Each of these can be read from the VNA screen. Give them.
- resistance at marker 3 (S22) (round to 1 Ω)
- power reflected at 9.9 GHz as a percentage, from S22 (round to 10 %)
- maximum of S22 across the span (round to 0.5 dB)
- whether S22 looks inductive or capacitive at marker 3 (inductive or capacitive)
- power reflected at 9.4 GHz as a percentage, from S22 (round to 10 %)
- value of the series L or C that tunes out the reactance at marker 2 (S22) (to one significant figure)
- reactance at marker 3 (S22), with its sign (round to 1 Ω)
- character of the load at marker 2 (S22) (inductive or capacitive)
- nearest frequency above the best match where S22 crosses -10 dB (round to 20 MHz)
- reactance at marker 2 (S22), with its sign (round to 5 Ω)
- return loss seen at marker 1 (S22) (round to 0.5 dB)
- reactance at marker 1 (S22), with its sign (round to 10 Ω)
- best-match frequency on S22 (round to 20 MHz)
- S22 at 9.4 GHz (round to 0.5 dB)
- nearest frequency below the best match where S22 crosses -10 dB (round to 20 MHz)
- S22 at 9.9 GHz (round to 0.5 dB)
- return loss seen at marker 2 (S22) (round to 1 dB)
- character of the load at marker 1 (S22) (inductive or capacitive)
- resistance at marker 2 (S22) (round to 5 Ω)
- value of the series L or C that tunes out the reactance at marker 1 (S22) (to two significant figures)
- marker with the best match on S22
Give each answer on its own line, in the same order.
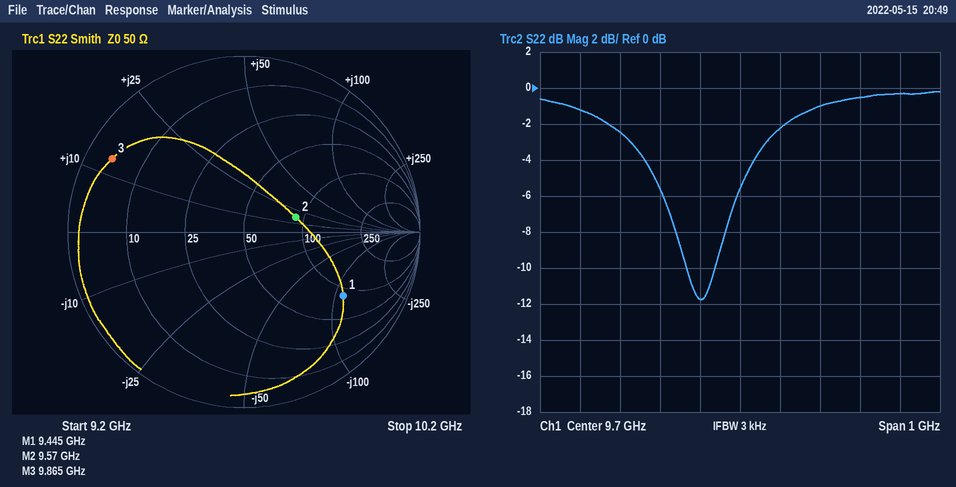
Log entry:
4 Ω
80 %
0.0 dB
inductive
60 %
1 pF
+13 Ω
inductive
9.64 GHz
+15 Ω
3.5 dB
-110 Ω
9.60 GHz
-2.5 dB
9.56 GHz
-1.0 dB
10 dB
capacitive
90 Ω
1.9 nH
marker 2
